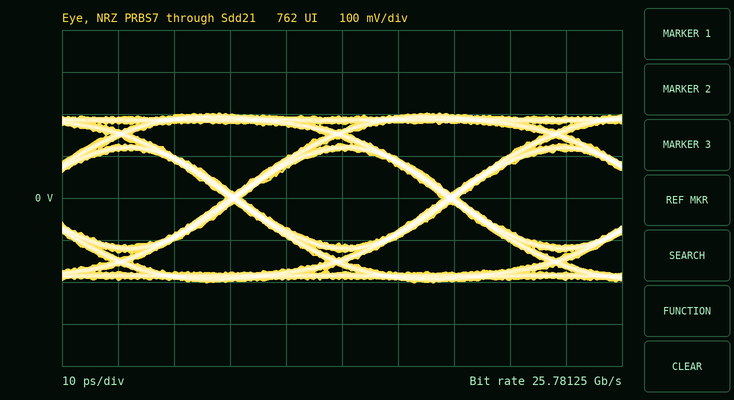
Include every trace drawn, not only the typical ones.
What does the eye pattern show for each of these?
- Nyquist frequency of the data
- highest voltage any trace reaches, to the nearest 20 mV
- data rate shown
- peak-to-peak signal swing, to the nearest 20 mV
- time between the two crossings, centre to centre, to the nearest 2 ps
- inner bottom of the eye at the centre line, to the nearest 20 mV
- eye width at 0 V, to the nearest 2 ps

12.89062 GHz
200 mV
25.78125 Gb/s
400 mV
38 ps
-120 mV
36 ps
